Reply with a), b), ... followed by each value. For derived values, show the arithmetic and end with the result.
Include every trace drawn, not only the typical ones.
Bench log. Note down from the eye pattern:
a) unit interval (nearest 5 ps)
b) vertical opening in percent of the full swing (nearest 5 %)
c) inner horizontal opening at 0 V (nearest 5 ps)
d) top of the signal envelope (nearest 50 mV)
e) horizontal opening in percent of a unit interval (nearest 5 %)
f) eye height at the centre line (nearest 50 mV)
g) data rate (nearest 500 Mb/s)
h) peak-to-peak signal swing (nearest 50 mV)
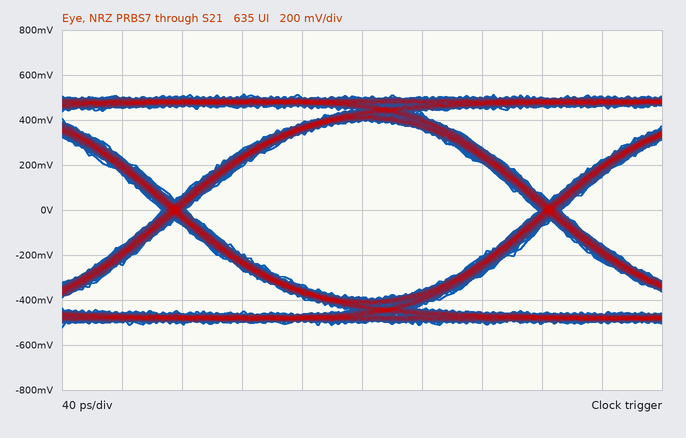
a) 250 ps
b) 800 mV / 1.05 V ≈ 76.2 %, so 75 % to the nearest 5 %
c) 235 ps
d) 500 mV
e) 235 ps / 250 ps ≈ 94.0 %, so 95 % to the nearest 5 %
f) 800 mV
g) 4.0 Gb/s
h) 1.05 V
